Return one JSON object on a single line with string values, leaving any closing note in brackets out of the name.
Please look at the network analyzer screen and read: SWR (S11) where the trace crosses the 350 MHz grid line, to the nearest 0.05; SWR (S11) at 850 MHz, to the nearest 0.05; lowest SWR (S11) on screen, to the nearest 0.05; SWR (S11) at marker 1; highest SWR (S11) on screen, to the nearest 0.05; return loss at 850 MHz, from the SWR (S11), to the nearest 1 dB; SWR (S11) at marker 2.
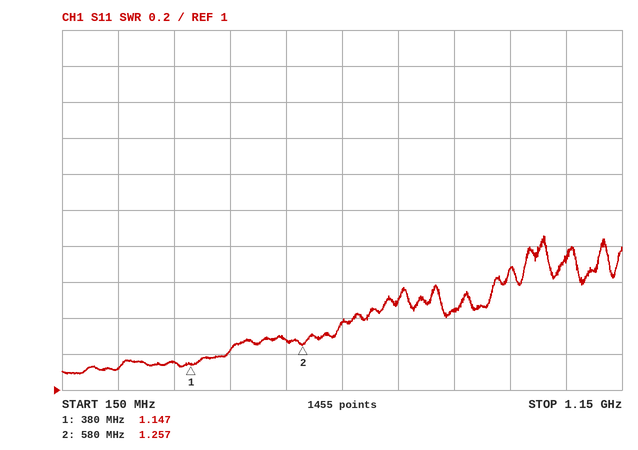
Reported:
{"SWR (S11) where the trace crosses the 350 MHz grid line, to the nearest 0.05": "1.15", "SWR (S11) at 850 MHz, to the nearest 0.05": "1.45", "lowest SWR (S11) on screen, to the nearest 0.05": "1.10", "SWR (S11) at marker 1": "1.147", "highest SWR (S11) on screen, to the nearest 0.05": "1.85", "return loss at 850 MHz, from the SWR (S11), to the nearest 1 dB": "15 dB", "SWR (S11) at marker 2": "1.257"}
